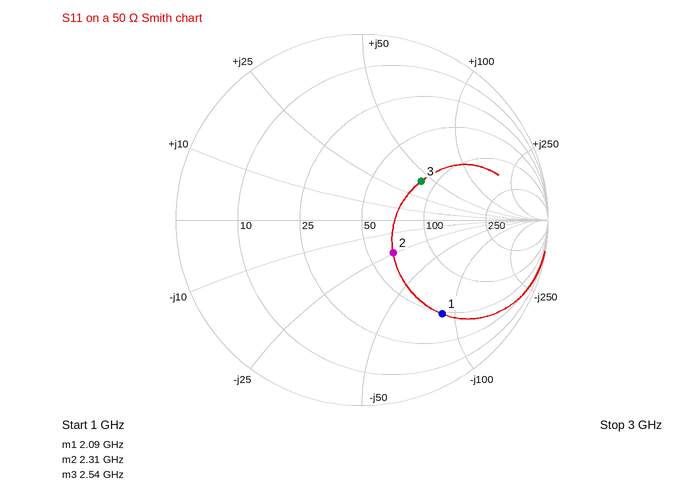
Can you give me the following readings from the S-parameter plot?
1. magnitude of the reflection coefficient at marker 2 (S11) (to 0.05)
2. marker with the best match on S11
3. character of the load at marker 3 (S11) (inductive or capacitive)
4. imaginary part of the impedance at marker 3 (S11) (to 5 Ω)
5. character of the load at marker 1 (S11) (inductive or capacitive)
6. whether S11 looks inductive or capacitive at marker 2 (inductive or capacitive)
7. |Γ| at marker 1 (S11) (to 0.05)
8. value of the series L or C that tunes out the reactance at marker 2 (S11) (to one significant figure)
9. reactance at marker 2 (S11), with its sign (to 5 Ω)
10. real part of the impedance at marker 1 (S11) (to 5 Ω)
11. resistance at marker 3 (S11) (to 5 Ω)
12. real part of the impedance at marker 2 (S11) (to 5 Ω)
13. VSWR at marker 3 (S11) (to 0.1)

0.25
marker 2
inductive
+40 Ω
capacitive
capacitive
0.65
2 nH
-25 Ω
50 Ω
85 Ω
65 Ω
2.2
